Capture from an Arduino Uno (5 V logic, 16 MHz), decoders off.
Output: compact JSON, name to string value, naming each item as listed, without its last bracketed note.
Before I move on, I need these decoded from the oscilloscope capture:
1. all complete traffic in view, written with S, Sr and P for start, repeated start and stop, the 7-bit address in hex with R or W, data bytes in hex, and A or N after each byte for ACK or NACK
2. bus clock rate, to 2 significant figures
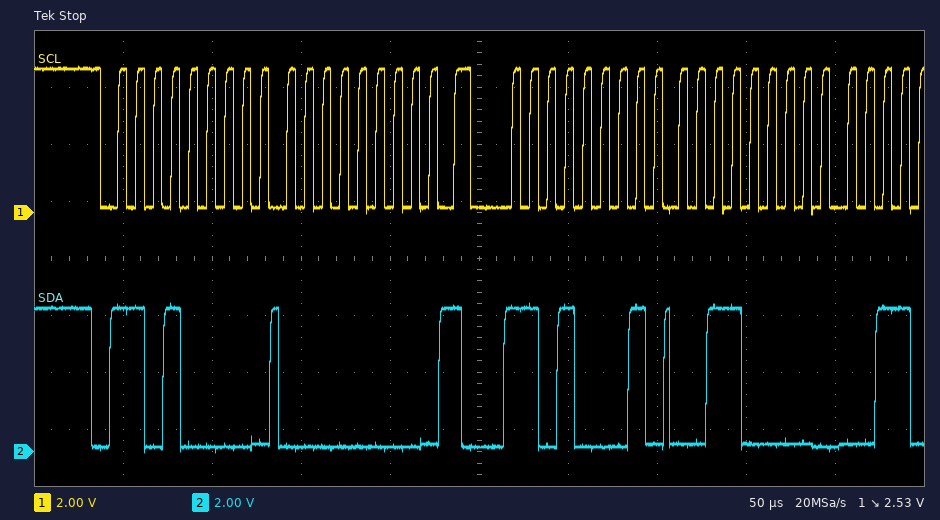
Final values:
{"all complete traffic in view, written with S, Sr and P for start, repeated start and stop, the 7-bit address in hex with R or W, data bytes in hex, and A or N after each byte for ACK or NACK": "S 68W A 00 A Sr 68R A 30 A", "bus clock rate, to 2 significant figures": "100 kHz"}
